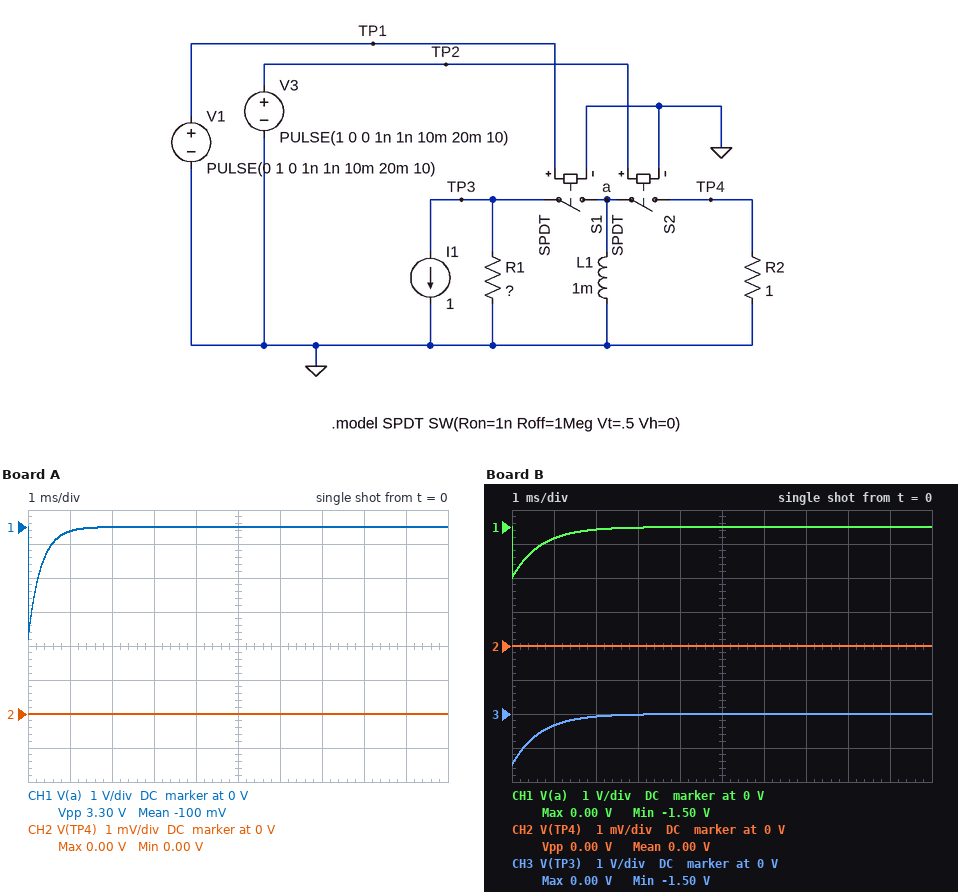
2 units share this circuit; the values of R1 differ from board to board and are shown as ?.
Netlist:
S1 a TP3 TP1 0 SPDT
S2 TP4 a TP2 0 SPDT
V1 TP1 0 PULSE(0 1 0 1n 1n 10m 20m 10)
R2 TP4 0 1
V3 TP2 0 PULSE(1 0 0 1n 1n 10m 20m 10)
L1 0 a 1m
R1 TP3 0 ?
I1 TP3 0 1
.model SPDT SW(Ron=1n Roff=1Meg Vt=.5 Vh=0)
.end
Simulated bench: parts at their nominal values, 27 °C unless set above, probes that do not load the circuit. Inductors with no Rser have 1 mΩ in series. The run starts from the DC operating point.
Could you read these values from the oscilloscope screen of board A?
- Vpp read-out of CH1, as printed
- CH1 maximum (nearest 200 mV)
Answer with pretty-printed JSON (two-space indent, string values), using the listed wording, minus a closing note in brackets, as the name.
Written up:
{
  "Vpp read-out of CH1, as printed": "3.30 V",
  "CH1 maximum": "0 V"
}
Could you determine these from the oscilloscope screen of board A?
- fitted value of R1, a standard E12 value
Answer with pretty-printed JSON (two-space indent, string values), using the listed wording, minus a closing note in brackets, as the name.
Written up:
{
  "fitted value of R1, a standard E12 value": "3.3 Ω"
}
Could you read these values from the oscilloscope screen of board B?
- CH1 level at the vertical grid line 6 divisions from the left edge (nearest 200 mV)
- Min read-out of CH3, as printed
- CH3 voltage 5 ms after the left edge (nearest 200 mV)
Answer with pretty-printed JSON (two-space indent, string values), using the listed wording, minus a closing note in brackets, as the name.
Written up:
{
  "CH1 level at the vertical grid line 6 divisions from the left edge": "0 V",
  "Min read-out of CH3, as printed": "-1.50 V",
  "CH3 voltage 5 ms after the left edge": "0 V"
}
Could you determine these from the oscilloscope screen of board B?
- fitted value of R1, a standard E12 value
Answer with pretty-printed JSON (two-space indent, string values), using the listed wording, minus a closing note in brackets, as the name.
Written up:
{
  "fitted value of R1, a standard E12 value": "1.5 Ω"
}
